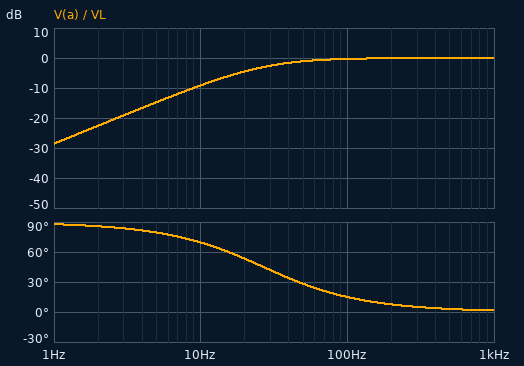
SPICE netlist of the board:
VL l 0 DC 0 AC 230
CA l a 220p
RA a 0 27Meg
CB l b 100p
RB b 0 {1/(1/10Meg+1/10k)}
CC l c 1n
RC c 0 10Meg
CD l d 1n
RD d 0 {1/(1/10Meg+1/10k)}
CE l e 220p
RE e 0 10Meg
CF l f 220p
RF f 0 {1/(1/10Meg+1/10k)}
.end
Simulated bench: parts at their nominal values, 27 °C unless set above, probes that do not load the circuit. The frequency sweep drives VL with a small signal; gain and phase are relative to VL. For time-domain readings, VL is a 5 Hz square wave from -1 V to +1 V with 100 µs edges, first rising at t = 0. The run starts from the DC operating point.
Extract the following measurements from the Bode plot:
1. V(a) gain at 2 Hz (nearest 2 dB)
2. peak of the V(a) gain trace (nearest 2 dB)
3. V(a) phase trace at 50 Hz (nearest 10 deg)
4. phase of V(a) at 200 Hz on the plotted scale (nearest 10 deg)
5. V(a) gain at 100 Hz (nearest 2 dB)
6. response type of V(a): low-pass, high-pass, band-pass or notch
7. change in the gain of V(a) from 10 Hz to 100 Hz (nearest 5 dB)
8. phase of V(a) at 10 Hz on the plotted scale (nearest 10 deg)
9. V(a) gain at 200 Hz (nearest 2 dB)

-22 dB
0 dB
30 deg
10 deg
0 dB
high-pass
10 dB
70 deg
0 dB
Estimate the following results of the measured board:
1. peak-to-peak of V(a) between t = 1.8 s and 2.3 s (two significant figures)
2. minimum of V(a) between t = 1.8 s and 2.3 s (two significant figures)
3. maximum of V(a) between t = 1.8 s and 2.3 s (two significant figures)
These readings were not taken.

4.0 V
-2.0 V
2.0 V
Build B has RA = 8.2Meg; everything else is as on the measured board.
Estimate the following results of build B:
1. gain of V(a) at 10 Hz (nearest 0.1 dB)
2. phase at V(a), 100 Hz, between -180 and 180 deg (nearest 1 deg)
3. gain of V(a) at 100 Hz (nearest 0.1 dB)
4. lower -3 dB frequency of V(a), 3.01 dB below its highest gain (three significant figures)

-19.0 dB
41 deg
-2.5 dB
88.2 Hz
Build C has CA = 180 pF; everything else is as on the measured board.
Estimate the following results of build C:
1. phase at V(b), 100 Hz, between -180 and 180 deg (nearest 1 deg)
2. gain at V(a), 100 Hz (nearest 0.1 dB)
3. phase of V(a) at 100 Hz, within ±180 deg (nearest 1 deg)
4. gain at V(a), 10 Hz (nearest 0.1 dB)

90 deg
-0.4 dB
18 deg
-10.7 dB
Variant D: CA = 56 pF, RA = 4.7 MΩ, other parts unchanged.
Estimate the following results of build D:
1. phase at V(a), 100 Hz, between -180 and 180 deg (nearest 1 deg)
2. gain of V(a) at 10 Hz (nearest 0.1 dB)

81 deg
-35.6 dB
